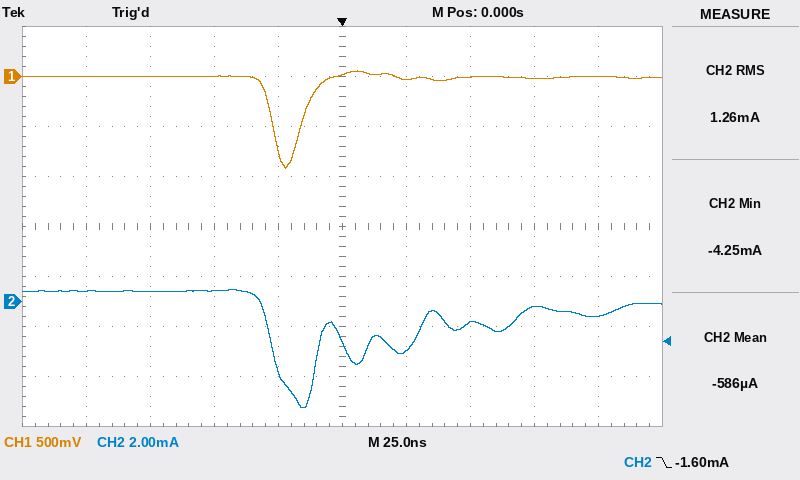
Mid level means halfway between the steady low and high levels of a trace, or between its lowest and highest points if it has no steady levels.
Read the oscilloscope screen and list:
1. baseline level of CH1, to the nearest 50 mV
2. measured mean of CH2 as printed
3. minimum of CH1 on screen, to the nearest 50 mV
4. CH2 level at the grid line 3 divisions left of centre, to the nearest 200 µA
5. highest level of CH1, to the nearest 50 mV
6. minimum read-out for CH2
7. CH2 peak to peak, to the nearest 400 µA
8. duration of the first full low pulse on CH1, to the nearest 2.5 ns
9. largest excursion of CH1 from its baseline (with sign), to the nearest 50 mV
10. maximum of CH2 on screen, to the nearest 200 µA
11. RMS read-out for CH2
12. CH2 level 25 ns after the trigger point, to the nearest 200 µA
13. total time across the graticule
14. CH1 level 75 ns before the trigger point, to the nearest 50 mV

0 mV
-586 µA
-900 mV
400 µA
50 mV
-4.25 mA
4.8 mA
12.5 ns
-900 mV
400 µA
1.26 mA
-2.0 mA
250 ns
0 mV
